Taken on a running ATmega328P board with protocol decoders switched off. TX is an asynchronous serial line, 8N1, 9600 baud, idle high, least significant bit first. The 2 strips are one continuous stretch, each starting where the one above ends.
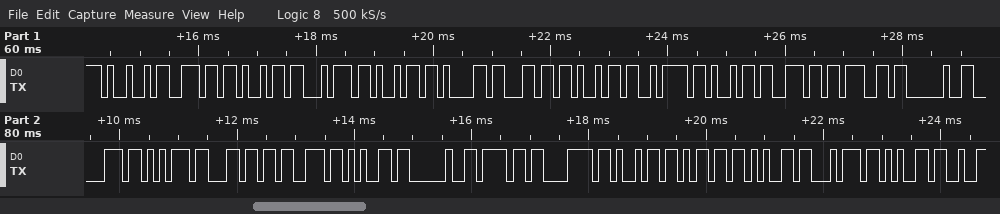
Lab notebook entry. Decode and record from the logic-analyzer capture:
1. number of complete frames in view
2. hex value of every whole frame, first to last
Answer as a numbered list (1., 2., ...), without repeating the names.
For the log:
1. 26
2. 49 6E 69 74 69 61 6C 69 7A 69 6E 67 20 70 75 6C 73 65 20 6F 78 69 6D 65 74 65
